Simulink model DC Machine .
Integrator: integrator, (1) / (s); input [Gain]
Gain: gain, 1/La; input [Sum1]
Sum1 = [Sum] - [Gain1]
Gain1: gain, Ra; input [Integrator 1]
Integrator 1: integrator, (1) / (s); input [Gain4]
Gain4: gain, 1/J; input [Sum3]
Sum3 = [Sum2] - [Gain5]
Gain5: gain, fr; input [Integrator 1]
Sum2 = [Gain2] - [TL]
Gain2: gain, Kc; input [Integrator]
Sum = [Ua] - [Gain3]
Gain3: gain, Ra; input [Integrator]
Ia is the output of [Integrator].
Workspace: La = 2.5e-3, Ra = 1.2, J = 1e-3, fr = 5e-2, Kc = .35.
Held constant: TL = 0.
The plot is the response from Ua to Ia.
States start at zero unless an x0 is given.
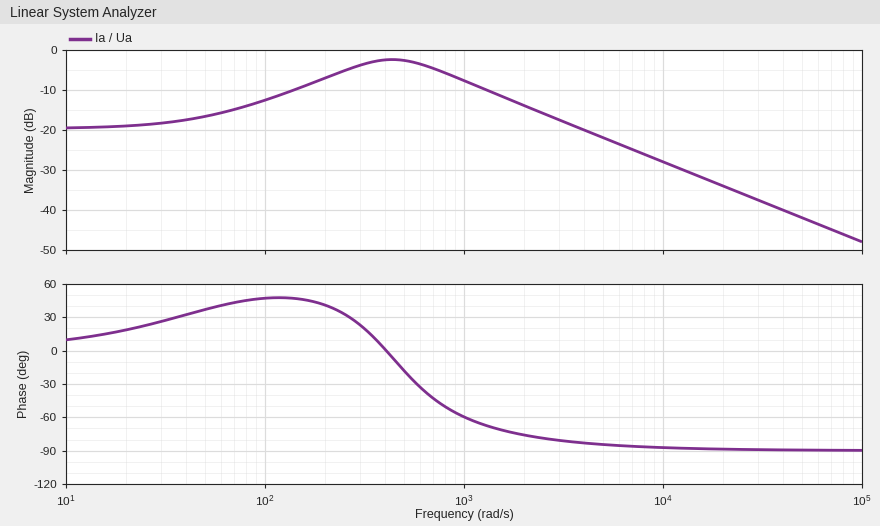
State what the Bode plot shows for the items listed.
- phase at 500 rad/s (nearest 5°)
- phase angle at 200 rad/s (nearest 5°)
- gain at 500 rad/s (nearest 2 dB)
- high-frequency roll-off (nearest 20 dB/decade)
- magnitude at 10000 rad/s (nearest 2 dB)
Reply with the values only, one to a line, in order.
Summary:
-20°
40°
-2 dB
-20 dB/decade
-28 dB
